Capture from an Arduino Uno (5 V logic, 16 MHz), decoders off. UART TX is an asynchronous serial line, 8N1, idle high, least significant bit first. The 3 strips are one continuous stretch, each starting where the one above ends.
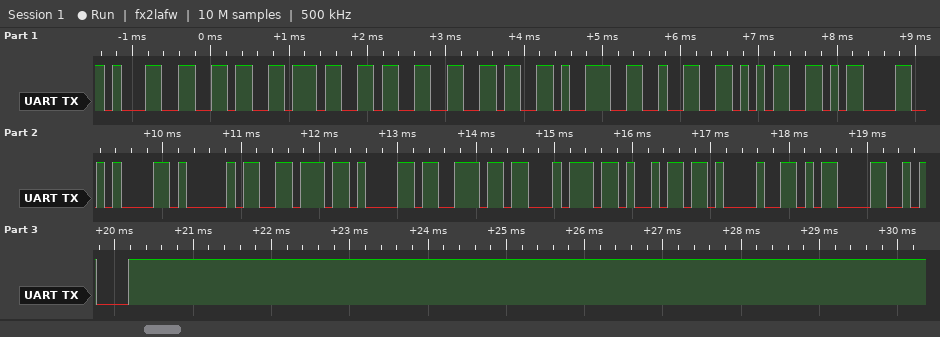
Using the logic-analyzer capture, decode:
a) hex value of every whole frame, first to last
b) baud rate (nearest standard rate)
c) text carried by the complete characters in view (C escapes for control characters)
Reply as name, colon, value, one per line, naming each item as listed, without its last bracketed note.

hex value of every whole frame, first to last: 31 36 37 33 36 39 32 35 0D 0A 41 76 61 6E 74 69 21 0D 0A
baud rate: 9600 baud
text carried by the complete characters in view: "16736925\r\nAvanti!\r\n"
